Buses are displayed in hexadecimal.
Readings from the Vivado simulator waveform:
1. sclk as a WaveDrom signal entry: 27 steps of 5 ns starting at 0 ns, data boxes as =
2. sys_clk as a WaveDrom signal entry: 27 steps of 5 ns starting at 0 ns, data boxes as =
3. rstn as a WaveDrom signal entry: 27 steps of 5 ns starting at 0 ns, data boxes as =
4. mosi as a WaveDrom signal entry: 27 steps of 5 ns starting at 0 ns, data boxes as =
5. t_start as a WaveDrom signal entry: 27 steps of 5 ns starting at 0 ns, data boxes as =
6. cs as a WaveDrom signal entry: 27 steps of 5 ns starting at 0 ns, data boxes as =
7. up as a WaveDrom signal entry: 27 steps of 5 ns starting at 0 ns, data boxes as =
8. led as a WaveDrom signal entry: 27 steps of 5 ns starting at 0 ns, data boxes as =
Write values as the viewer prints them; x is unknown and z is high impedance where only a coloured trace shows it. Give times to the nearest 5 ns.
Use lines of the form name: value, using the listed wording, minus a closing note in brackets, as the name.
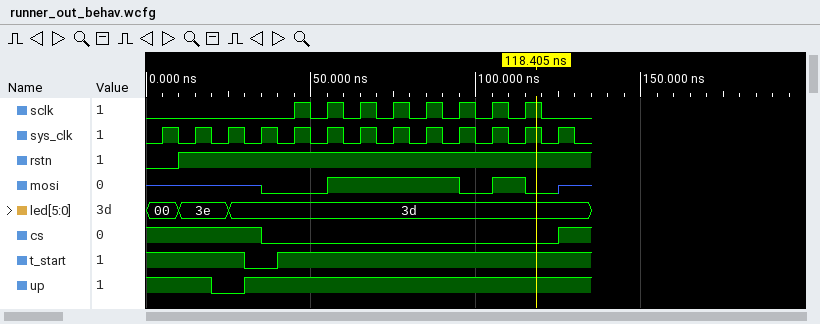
sclk as a WaveDrom signal entry: 27 steps of 5 ns starting at 0 ns, data boxes as =: {name: 'sclk', wave: '0........1010101010101010..'}
sys_clk as a WaveDrom signal entry: 27 steps of 5 ns starting at 0 ns, data boxes as =: {name: 'sys_clk', wave: '010101010101010101010101010'}
rstn as a WaveDrom signal entry: 27 steps of 5 ns starting at 0 ns, data boxes as =: {name: 'rstn', wave: '0.1........................'}
mosi as a WaveDrom signal entry: 27 steps of 5 ns starting at 0 ns, data boxes as =: {name: 'mosi', wave: 'z......0...1.......0.1.0.z.'}
t_start as a WaveDrom signal entry: 27 steps of 5 ns starting at 0 ns, data boxes as =: {name: 't_start', wave: '1.....0.1..................'}
cs as a WaveDrom signal entry: 27 steps of 5 ns starting at 0 ns, data boxes as =: {name: 'cs', wave: '1......0.................1.'}
up as a WaveDrom signal entry: 27 steps of 5 ns starting at 0 ns, data boxes as =: {name: 'up', wave: '1...0.1....................'}
led as a WaveDrom signal entry: 27 steps of 5 ns starting at 0 ns, data boxes as =: {name: 'led', wave: '=.=..=.....................', data: '00 3e 3d'}
